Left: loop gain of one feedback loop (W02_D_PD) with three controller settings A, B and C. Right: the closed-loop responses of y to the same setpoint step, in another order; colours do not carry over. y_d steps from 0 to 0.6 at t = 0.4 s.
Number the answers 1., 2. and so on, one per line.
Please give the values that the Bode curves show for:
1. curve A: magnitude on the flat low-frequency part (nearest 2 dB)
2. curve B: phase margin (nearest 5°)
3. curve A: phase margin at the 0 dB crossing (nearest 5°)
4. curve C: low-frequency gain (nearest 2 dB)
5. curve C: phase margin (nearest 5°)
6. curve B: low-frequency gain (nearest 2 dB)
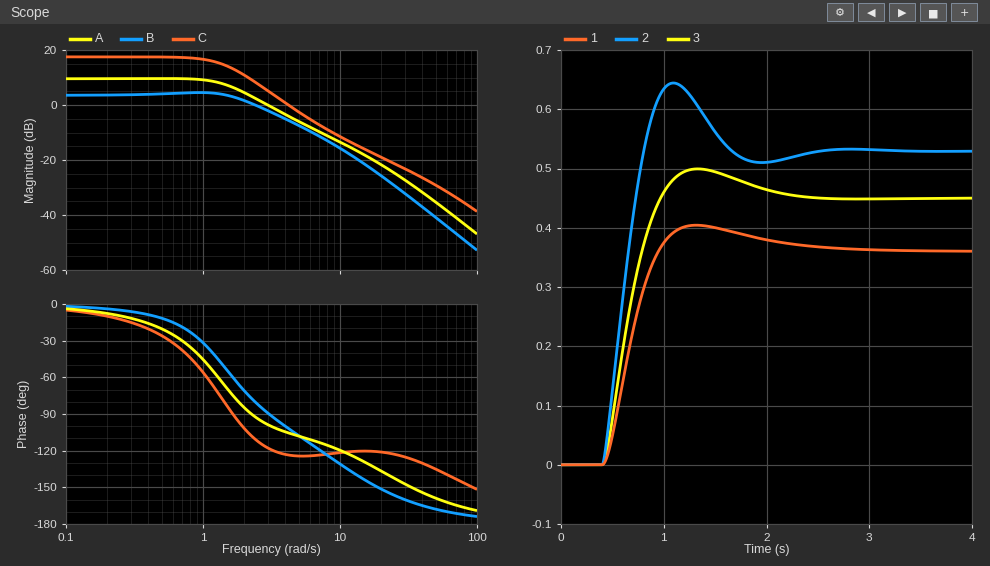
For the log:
1. 10 dB
2. 100°
3. 80°
4. 18 dB
5. 55°
6. 4 dB
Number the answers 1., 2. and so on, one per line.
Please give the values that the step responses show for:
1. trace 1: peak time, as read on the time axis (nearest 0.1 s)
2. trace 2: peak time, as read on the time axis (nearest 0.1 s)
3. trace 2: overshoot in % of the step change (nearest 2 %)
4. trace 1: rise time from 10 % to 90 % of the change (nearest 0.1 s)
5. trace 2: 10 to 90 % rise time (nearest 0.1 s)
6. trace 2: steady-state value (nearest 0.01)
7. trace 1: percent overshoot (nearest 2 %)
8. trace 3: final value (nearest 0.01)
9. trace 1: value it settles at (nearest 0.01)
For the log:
1. 1.3 s
2. 1.1 s
3. 22 %
4. 0.4 s
5. 0.3 s
6. 0.53
7. 12 %
8. 0.45
9. 0.36
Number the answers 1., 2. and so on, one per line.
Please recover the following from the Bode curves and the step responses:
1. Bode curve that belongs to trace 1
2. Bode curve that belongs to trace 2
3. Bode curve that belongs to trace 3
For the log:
1. B
2. C
3. A
